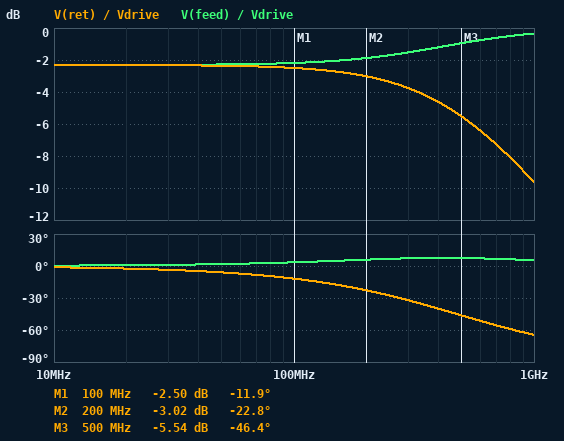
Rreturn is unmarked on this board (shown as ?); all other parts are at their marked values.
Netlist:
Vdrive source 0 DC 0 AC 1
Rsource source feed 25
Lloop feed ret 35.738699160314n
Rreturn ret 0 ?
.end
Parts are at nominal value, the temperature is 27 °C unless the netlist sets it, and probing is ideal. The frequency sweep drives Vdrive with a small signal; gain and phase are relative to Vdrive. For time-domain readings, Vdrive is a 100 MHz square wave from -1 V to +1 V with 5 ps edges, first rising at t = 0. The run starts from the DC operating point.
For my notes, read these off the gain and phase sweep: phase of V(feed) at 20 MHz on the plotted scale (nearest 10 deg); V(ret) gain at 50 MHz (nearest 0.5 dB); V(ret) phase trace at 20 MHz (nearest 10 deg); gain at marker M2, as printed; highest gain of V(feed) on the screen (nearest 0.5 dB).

0 deg
-2.5 dB
0 deg
-3.02 dB
-0.5 dB
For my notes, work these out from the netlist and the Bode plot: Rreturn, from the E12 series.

82 Ω
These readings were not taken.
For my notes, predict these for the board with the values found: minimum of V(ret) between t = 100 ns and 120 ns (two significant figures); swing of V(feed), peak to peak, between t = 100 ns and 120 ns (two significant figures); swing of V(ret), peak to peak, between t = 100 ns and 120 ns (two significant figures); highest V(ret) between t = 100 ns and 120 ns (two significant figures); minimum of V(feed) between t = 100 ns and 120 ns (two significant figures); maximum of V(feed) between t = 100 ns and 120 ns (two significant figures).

-770 mV
2.5 V
1.5 V
770 mV
-1.2 V
1.2 V
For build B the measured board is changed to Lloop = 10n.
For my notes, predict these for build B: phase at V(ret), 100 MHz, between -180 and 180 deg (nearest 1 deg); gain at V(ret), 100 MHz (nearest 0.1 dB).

-3 deg
-2.3 dB
